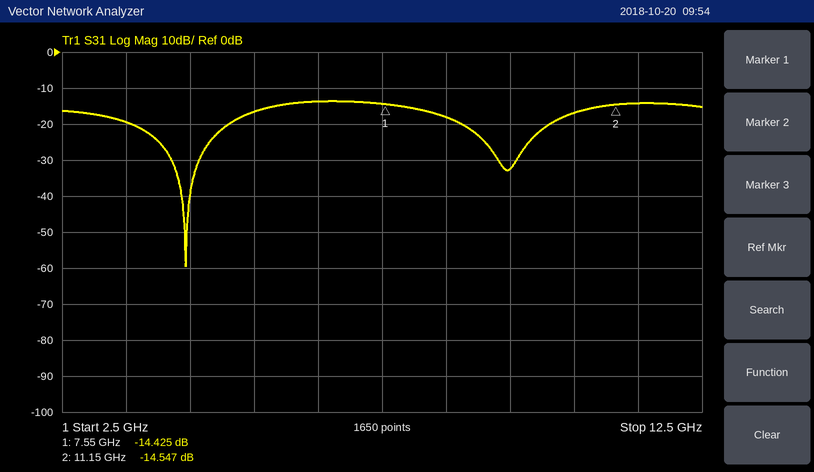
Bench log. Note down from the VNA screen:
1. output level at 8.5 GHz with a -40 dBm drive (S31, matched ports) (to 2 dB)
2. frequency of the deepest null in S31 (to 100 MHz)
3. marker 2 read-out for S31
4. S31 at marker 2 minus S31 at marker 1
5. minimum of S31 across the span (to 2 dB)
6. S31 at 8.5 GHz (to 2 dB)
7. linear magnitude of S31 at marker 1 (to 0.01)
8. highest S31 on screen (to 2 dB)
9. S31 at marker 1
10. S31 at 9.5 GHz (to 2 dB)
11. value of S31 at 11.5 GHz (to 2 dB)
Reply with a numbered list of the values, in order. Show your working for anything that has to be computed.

1. -40 dBm + (-18 dB) = -58 dBm
2. 4.4 GHz
3. -14.547 dB
4. -14.547 − (-14.425) = -0.122 dB
5. -60 dB
6. -18 dB
7. 10^(-14.425/20) ≈ 0.19
8. -14 dB
9. -14.425 dB
10. -32 dB
11. -14 dB
